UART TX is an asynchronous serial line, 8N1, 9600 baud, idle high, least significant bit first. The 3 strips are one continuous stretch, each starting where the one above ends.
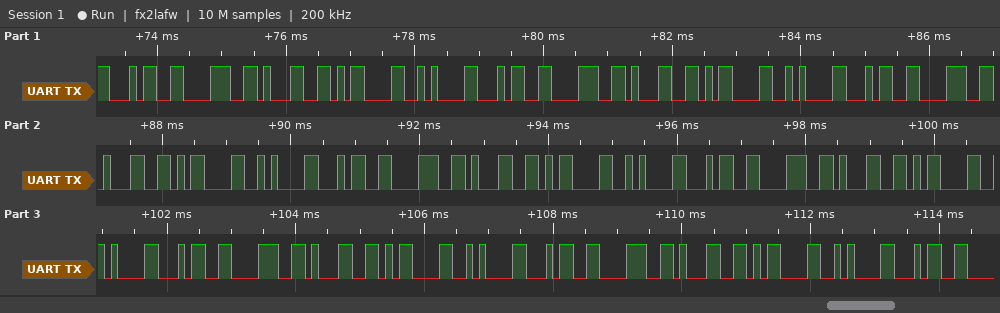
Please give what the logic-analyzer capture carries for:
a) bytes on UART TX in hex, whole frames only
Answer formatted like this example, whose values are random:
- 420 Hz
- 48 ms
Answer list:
- 34 38 31 0D 0A 34 38 31 0D 0A 34 38 31 0D 0A 34 38 31 0D 0A 34 38 31 0D 0A 34 38 31 0D 0A 34 38 31 0D 0A 34
